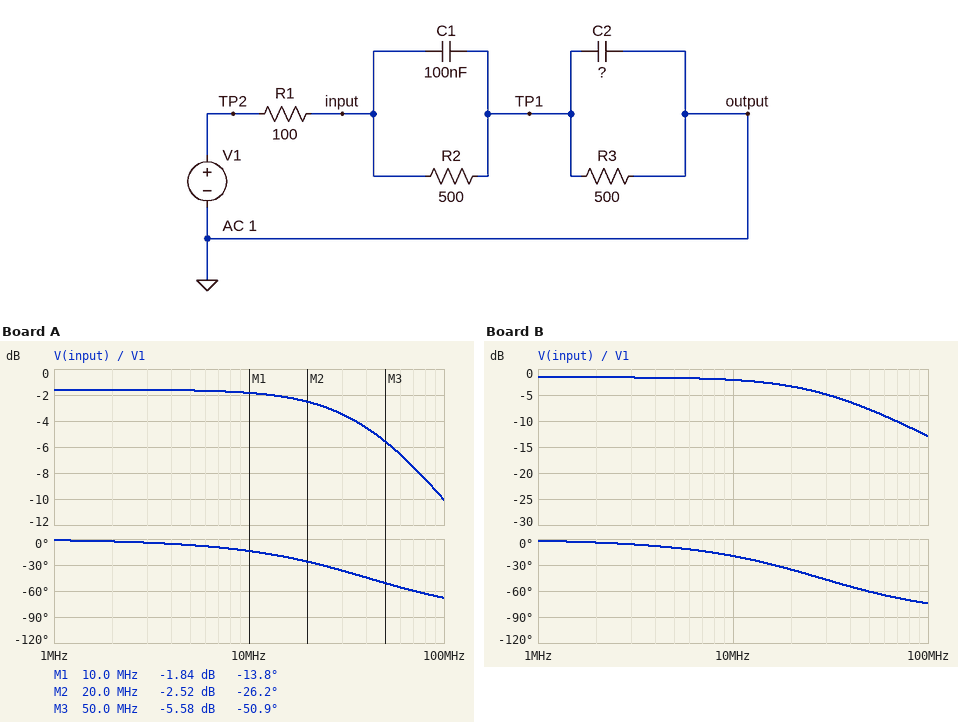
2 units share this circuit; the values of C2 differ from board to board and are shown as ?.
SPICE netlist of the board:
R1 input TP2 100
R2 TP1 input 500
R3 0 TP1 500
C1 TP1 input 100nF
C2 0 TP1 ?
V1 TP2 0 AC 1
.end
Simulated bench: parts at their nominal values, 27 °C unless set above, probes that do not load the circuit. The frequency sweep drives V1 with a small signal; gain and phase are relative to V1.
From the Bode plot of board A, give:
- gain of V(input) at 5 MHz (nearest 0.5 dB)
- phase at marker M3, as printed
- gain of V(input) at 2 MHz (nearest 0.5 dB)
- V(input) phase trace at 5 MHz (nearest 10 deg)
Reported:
-1.5 dB
-50.9 deg
-1.5 dB
-10 deg
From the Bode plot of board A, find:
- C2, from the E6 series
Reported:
47 pF
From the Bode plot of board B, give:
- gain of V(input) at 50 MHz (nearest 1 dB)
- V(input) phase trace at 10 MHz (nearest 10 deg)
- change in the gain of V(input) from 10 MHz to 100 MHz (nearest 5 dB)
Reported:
-8 dB
-20 deg
-10 dB
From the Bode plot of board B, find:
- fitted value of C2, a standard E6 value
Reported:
68 pF
